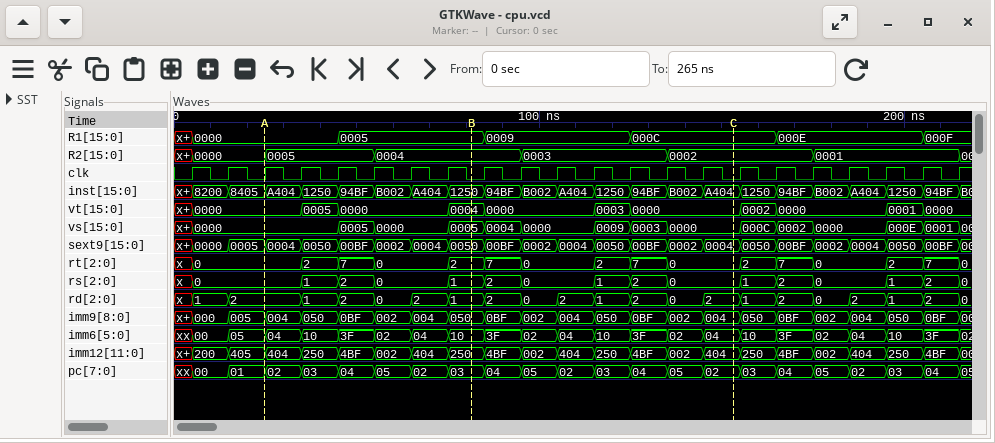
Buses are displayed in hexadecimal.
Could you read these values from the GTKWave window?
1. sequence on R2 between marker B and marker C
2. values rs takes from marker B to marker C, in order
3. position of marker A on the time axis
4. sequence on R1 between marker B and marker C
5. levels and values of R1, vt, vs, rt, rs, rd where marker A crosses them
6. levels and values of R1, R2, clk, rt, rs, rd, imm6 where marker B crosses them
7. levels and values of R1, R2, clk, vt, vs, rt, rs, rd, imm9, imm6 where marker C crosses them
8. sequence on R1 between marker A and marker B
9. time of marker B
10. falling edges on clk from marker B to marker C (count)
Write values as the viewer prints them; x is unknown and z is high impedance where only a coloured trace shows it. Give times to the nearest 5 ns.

0004, 0003, 0002
1, 2, 0, 1, 2, 0
25 ns
0005, 0009, 000C
R1=0000, vt=0000, vs=0000, rt=0, rs=0, rd=2
R1=0005, R2=0004, clk=0, rt=2, rs=1, rd=1, imm6=10
R1=000C, R2=0002, clk=0, vt=0000, vs=0000, rt=0, rs=0, rd=2, imm9=004, imm6=04
0000, 0005
80 ns
7
